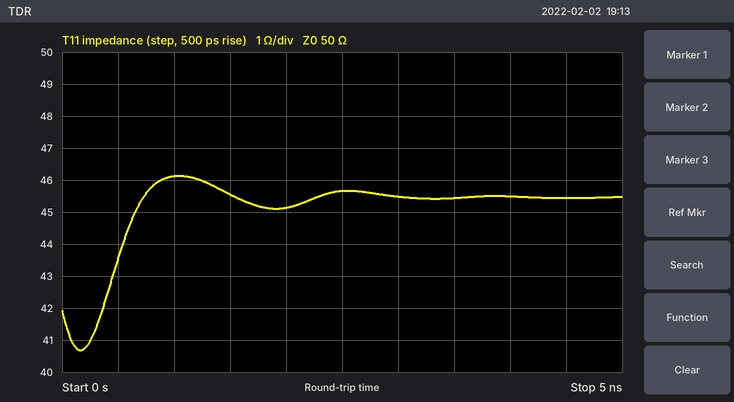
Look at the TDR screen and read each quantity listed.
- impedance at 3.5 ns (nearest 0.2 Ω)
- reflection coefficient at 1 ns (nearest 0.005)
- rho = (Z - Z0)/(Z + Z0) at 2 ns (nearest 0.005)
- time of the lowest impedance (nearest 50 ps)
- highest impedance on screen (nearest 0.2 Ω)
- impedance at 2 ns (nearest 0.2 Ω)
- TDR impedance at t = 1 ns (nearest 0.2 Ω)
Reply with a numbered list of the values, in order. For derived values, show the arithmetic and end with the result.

1. 45.4 Ω
2. (46.2 − 50)/(46.2 + 50) ≈ -0.040
3. (45.2 − 50)/(45.2 + 50) ≈ -0.050
4. 150 ps
5. 46.2 Ω
6. 45.2 Ω
7. 46.2 Ω
